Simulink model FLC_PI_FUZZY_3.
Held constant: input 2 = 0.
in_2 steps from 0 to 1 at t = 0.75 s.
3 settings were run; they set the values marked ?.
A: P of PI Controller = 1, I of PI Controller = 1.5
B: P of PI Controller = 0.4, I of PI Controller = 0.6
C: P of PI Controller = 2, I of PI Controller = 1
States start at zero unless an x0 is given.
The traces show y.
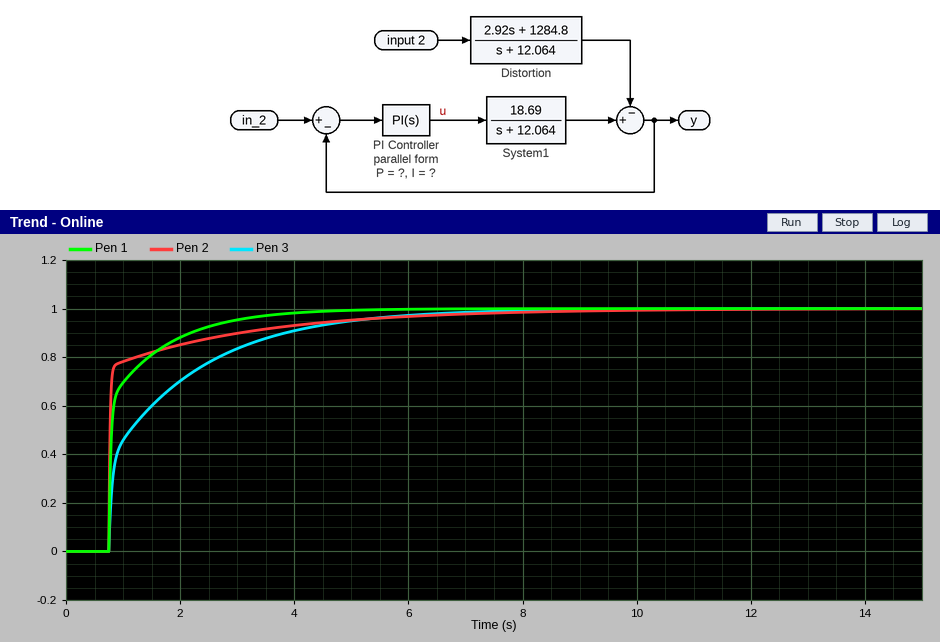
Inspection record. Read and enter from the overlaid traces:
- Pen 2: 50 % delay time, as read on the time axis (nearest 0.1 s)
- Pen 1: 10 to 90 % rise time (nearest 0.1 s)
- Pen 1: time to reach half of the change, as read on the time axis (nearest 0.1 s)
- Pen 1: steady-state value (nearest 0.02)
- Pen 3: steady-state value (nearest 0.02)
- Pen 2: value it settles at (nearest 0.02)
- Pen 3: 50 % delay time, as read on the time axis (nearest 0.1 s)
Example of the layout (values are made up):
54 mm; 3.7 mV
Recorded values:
0.8 s; 1.4 s; 0.8 s; 1.00; 1.00; 1.00; 1.1 s
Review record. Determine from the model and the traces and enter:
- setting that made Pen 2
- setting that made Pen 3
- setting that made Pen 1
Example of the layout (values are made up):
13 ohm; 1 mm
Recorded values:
C; B; A
